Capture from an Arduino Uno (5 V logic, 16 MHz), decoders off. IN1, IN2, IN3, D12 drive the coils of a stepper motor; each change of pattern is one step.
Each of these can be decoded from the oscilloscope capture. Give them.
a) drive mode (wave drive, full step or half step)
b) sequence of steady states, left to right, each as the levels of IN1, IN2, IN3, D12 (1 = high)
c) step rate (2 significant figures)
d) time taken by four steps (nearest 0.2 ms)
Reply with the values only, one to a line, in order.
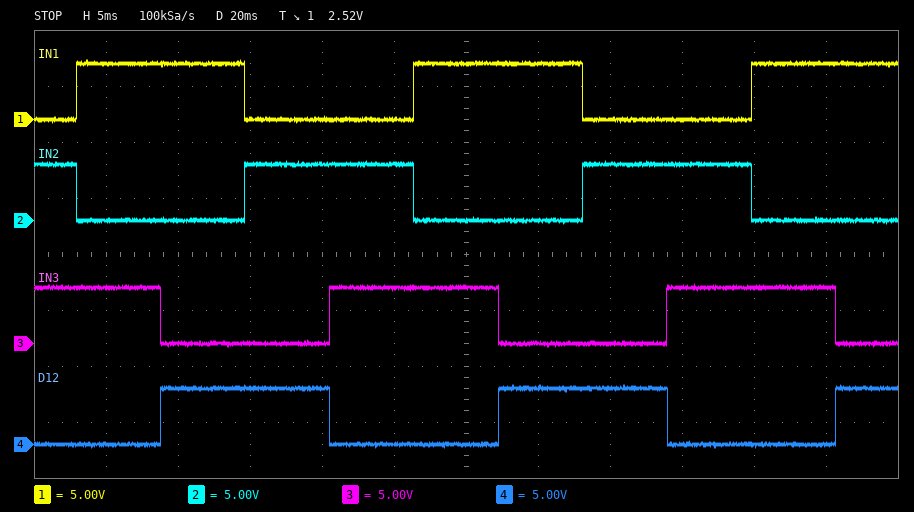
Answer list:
full step
0110 1010 1001 0101 0110 1010 1001 0101 0110 1010 1001
170 steps/s
23.4 ms
